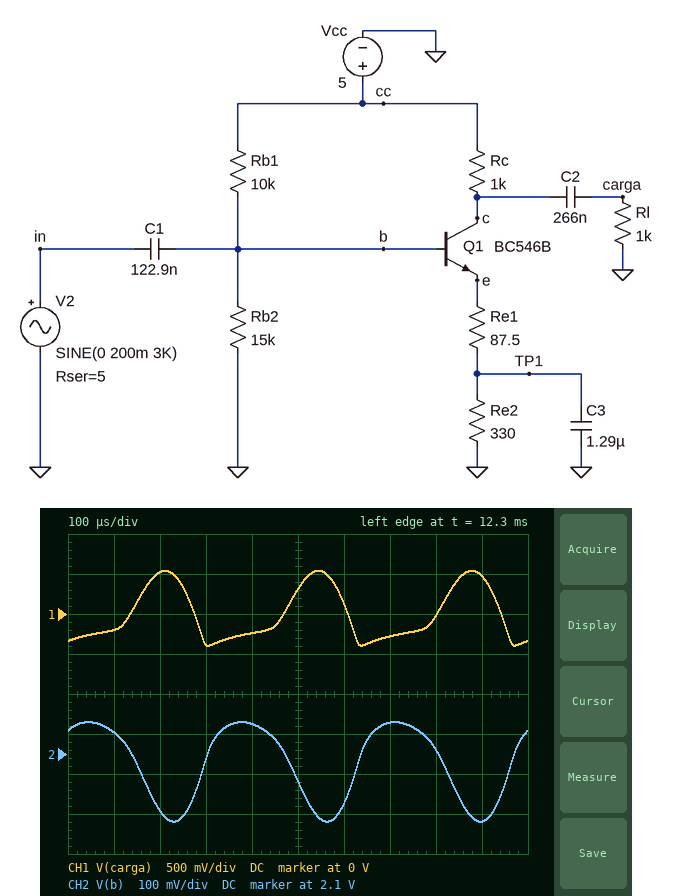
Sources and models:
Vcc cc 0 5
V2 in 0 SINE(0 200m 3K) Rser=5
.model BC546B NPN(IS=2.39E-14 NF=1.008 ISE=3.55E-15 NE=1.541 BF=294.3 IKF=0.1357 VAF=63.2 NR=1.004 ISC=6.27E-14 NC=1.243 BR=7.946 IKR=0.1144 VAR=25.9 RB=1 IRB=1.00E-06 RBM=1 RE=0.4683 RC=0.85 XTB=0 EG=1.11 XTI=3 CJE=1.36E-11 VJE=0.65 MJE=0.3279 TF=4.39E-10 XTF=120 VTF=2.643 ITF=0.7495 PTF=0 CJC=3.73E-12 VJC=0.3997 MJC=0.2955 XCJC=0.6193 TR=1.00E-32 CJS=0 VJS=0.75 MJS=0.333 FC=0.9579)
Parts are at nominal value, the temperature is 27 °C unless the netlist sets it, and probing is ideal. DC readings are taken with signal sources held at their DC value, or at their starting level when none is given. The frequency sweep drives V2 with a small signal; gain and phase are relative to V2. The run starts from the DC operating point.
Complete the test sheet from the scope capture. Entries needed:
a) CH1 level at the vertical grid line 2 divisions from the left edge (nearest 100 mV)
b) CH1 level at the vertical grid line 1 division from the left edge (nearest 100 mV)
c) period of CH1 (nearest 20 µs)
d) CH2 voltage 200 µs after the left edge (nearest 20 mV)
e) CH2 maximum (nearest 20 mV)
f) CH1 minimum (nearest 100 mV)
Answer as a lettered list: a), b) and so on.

a) 500 mV
b) -200 mV
c) 340 µs
d) 1.96 V
e) 2.18 V
f) -400 mV
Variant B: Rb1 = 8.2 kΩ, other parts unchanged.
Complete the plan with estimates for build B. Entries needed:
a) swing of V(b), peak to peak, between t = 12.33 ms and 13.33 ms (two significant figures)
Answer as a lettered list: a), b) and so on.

a) 210 mV
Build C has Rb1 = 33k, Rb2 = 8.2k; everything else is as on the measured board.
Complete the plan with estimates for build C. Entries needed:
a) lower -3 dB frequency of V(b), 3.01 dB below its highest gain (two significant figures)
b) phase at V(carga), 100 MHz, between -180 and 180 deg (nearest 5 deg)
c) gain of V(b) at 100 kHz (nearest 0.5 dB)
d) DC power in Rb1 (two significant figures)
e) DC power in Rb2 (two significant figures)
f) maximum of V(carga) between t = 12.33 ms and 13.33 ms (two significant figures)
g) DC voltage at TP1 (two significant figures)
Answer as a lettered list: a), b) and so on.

a) 210 Hz
b) 100 deg
c) 0 dB
d) 490 µW
e) 120 µW
f) 460 mV
g) 270 mV
